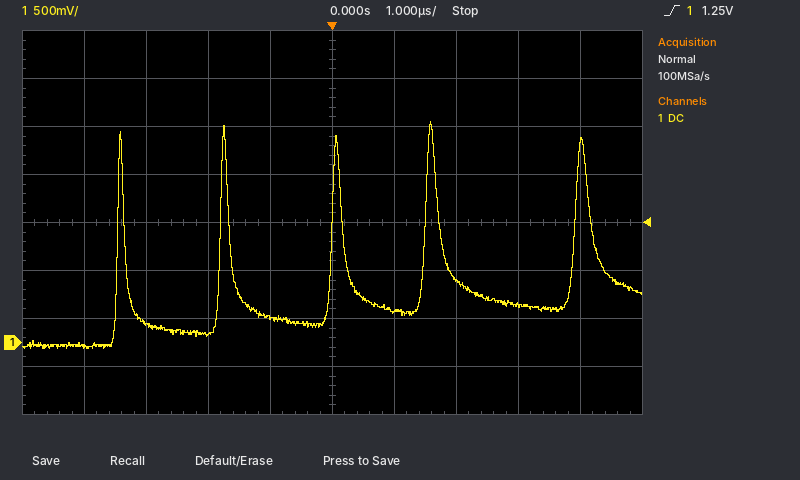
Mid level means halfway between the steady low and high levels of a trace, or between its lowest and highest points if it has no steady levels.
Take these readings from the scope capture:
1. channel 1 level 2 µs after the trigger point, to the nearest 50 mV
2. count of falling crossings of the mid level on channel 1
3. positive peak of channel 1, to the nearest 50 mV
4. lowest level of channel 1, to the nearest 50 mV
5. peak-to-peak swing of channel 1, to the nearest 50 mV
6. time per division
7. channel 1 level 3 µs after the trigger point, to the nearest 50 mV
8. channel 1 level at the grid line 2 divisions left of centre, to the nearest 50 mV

650 mV
5
2.30 V
-50 mV
2.35 V
1 µs
400 mV
100 mV
